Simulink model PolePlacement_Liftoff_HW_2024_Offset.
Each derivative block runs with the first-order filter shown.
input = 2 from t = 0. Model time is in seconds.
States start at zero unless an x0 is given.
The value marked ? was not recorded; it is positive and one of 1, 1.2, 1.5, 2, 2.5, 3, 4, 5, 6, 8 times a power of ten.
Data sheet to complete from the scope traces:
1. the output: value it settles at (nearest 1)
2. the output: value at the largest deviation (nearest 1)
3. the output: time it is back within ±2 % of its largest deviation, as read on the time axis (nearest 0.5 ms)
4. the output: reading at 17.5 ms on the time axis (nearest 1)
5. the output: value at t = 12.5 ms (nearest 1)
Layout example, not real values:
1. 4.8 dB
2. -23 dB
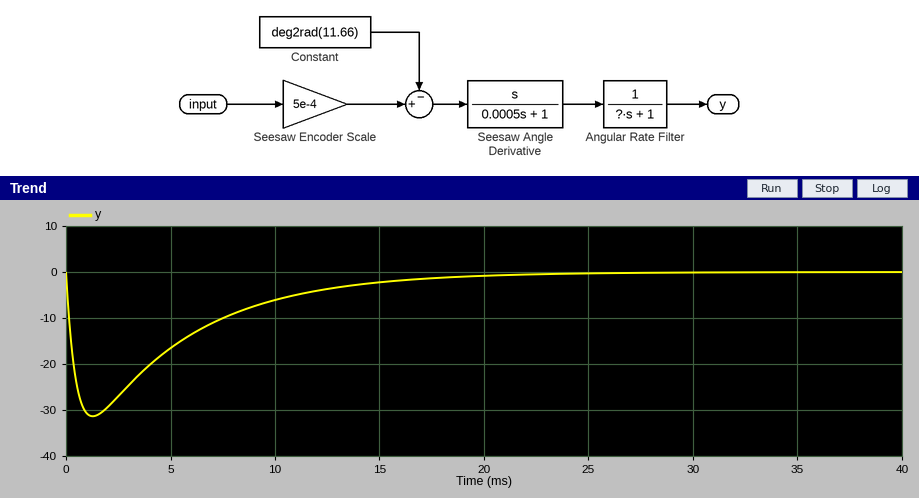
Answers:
1. 0
2. -31
3. 21.5 ms
4. -1
5. -4
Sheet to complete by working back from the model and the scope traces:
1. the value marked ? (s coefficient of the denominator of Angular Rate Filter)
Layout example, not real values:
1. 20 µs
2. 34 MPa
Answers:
1. 0.005
